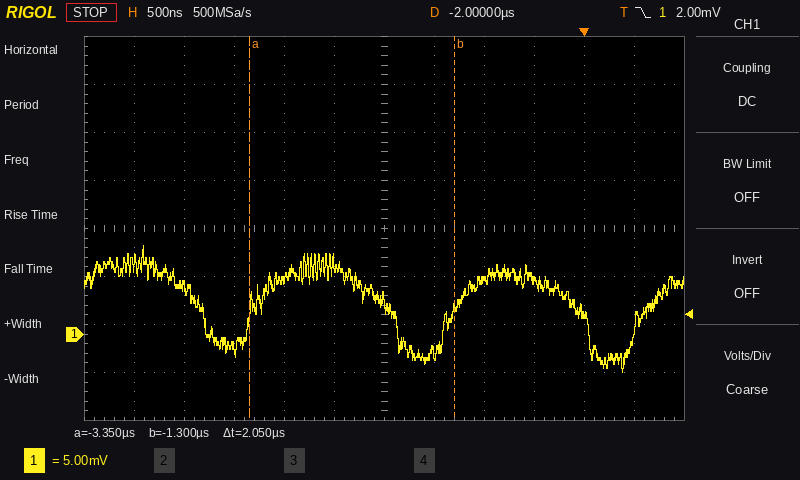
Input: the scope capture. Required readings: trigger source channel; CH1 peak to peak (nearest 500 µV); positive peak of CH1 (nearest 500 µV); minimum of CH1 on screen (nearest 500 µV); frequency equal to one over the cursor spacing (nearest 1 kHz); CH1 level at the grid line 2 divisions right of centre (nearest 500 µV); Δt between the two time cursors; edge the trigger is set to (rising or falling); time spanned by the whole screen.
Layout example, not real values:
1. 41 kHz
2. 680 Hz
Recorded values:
1. CH1
2. 13.0 mV
3. 9.0 mV
4. -4.0 mV
5. 488 kHz
6. 5.5 mV
7. 2.05 µs
8. falling
9. 6 µs
